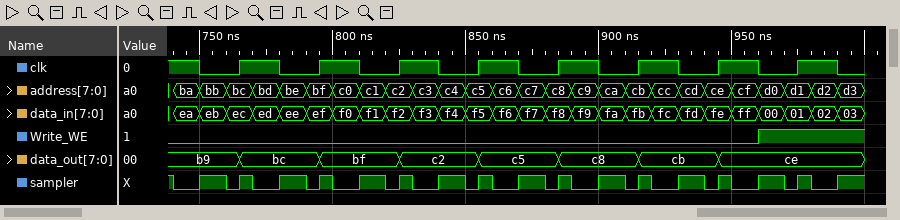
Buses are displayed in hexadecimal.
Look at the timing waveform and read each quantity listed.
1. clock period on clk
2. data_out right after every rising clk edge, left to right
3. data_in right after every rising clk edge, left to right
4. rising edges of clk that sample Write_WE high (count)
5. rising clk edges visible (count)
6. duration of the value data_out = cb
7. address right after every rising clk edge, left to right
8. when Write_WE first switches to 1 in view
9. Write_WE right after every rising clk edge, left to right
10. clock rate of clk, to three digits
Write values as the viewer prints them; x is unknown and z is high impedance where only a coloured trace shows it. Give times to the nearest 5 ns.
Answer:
30 ns
bc, bf, c2, c5, c8, cb, ce, ce
ec, ef, f2, f5, f8, fb, fe, 01
1
8
30 ns
bc, bf, c2, c5, c8, cb, ce, d1
960 ns
0 0 0 0 0 0 0 1
33.3 MHz
